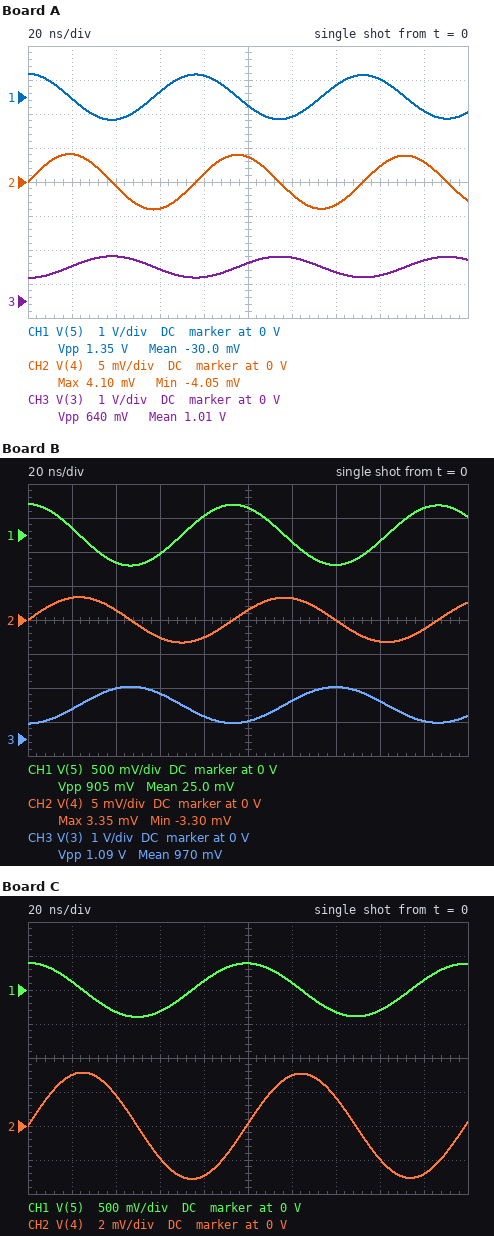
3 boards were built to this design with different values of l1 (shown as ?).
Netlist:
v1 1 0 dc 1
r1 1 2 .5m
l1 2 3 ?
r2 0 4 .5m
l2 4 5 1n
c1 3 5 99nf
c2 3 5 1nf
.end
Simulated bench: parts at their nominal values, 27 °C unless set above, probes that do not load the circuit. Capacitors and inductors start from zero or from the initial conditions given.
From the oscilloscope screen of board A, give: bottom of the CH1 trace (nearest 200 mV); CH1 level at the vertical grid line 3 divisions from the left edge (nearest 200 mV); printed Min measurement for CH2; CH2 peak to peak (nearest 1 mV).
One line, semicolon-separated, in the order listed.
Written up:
-600 mV; 200 mV; -4.05 mV; 8 mV
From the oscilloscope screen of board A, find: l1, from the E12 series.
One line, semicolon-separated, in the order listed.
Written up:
470 pH
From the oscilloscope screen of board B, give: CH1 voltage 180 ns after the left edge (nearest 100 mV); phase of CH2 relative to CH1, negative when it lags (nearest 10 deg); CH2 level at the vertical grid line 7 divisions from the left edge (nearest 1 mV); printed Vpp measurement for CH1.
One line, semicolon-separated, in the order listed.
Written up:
400 mV; -90 deg; 0 V; 905 mV
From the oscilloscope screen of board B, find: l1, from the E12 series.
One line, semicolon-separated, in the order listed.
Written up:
1.2 nH
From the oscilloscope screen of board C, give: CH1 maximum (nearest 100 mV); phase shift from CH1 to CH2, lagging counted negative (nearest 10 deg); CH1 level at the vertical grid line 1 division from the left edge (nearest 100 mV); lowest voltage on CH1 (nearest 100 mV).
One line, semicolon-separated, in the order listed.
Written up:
400 mV; -90 deg; 100 mV; -400 mV
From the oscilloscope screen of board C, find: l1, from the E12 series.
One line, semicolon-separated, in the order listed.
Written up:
1.5 nH
